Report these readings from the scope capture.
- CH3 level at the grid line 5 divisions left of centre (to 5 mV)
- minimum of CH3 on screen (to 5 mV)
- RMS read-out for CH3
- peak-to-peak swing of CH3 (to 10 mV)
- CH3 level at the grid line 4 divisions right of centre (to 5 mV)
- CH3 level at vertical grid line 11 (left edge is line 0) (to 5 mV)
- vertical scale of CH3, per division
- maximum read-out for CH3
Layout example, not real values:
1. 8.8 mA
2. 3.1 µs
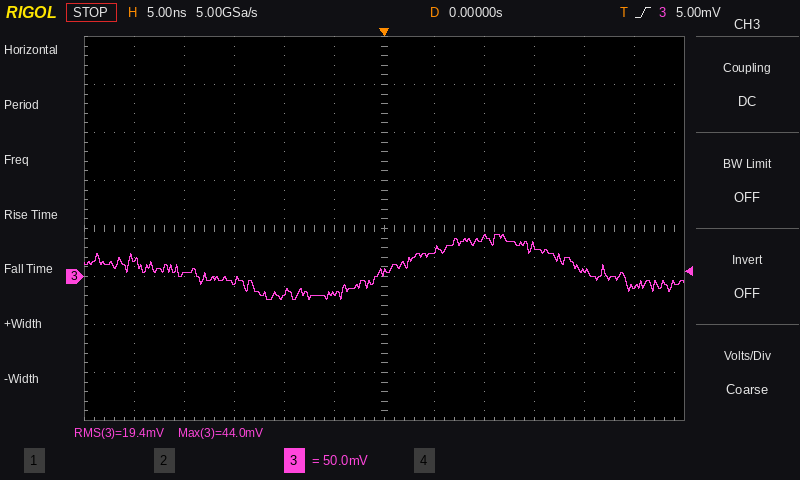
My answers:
1. 20 mV
2. -25 mV
3. 19.4 mV
4. 70 mV
5. 5 mV
6. -10 mV
7. 50 mV
8. 44.0 mV
